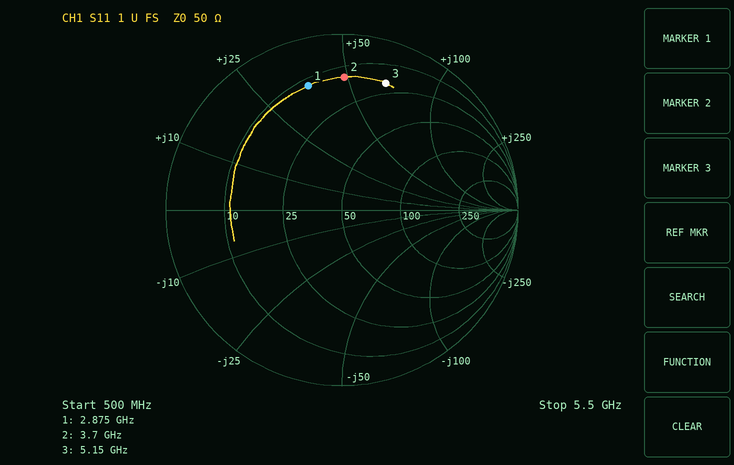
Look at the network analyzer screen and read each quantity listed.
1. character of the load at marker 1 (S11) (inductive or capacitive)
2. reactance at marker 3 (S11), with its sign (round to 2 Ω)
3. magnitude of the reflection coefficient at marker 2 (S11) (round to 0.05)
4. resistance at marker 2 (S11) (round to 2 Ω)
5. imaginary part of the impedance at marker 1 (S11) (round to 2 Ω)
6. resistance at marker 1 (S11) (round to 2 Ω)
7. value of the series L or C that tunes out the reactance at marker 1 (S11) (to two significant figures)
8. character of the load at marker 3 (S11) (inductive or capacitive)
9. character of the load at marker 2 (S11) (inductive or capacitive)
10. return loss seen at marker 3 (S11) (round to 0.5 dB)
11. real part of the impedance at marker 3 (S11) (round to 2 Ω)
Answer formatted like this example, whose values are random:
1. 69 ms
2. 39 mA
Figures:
1. inductive
2. +66 Ω
3. 0.75
4. 14 Ω
5. +36 Ω
6. 12 Ω
7. 1.5 pF
8. inductive
9. inductive
10. 2.5 dB
11. 20 Ω
